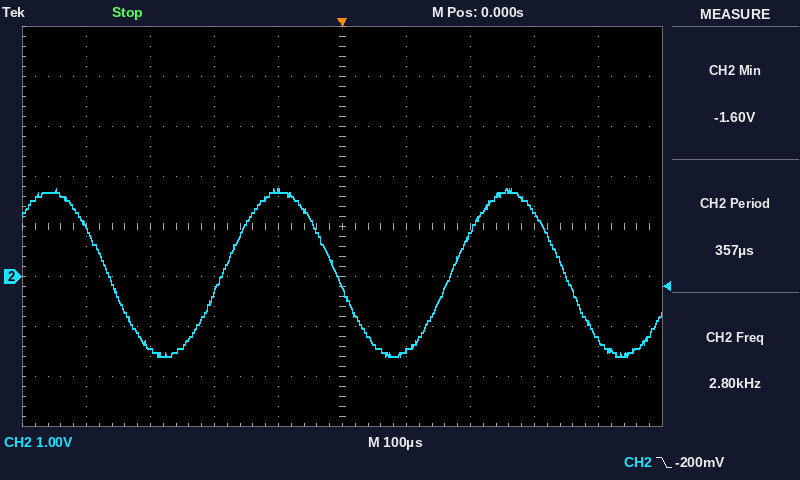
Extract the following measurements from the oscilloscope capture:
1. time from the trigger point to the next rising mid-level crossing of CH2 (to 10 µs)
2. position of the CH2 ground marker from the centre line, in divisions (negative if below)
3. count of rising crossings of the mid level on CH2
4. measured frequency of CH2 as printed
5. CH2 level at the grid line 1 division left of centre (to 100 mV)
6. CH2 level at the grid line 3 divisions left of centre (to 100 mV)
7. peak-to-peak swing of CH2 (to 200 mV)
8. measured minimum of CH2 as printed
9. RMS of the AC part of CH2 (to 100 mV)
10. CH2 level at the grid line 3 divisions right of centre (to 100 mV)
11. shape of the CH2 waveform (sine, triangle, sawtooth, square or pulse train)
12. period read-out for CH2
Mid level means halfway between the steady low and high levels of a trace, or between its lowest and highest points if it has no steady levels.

170 µs
-1.0 div
2
2.80 kHz
1.7 V
-1.5 V
3.4 V
-1.60 V
1.2 V
1.3 V
sine
357 µs
